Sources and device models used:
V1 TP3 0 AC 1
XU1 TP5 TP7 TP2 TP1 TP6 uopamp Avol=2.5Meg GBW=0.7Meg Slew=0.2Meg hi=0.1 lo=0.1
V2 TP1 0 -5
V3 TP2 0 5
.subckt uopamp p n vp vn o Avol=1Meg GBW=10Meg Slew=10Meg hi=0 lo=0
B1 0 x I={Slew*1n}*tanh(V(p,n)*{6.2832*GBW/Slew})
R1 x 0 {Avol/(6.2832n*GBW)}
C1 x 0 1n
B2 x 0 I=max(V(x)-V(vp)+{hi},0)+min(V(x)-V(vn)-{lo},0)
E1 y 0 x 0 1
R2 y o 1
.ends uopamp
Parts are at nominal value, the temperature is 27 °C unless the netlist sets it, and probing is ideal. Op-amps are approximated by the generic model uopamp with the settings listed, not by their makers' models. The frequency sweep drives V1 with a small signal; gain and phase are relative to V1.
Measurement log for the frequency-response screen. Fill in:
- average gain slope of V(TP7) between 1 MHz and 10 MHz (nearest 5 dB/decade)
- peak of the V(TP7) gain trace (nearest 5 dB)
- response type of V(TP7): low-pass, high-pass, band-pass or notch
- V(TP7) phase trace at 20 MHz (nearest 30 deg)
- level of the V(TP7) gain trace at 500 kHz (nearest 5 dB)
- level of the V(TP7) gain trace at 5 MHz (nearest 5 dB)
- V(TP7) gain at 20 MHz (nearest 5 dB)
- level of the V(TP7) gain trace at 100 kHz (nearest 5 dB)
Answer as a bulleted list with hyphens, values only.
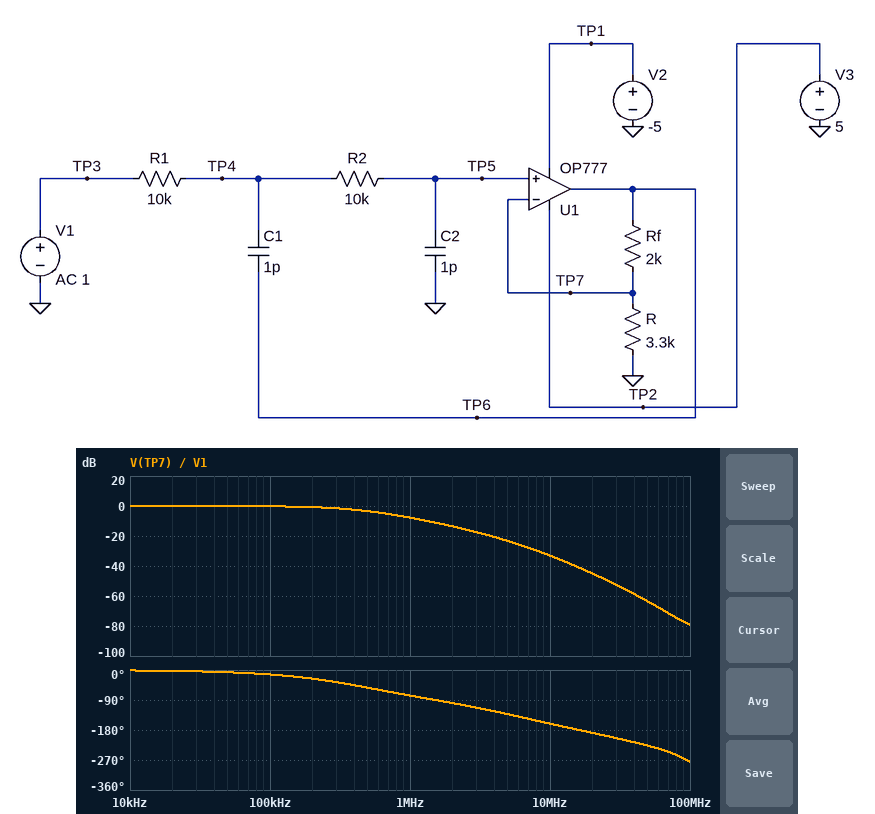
- -25 dB/decade
- 0 dB
- low-pass
- -180 deg
- -5 dB
- -25 dB
- -45 dB
- 0 dB
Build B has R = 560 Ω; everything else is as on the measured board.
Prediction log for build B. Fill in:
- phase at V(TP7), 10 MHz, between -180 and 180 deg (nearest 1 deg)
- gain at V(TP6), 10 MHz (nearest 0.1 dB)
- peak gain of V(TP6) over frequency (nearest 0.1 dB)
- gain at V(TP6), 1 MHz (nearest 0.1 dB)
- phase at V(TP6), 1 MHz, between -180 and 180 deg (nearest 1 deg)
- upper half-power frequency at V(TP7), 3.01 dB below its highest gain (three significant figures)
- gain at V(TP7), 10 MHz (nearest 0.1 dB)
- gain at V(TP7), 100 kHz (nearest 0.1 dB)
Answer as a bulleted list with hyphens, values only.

- -163 deg
- -29.0 dB
- 13.2 dB
- -2.9 dB
- -92 deg
- 160 kHz
- -42.2 dB
- -1.4 dB
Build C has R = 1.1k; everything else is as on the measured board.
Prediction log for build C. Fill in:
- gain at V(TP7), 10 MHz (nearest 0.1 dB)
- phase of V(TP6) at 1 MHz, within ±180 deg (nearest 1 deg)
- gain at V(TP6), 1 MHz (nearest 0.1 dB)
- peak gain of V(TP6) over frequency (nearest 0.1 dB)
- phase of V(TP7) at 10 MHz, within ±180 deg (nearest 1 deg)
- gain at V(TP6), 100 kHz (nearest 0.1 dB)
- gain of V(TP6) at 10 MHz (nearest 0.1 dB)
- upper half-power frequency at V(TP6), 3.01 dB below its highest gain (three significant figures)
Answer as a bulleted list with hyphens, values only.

- -38.0 dB
- -87 deg
- -3.1 dB
- 9.0 dB
- -162 deg
- 8.4 dB
- -29.0 dB
- 260 kHz
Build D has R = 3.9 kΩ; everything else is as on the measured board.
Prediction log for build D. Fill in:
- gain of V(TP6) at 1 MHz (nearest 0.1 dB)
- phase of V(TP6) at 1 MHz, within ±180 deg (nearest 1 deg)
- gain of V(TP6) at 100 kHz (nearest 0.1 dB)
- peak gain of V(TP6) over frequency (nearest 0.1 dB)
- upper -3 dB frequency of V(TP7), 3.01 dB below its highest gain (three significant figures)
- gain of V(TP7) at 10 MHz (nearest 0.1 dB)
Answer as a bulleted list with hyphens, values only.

- -3.7 dB
- -75 deg
- 3.4 dB
- 3.6 dB
- 483 kHz
- -32.6 dB
